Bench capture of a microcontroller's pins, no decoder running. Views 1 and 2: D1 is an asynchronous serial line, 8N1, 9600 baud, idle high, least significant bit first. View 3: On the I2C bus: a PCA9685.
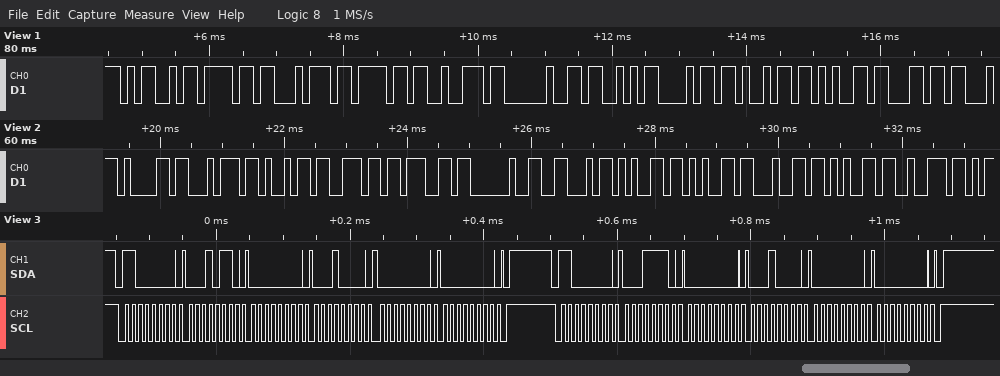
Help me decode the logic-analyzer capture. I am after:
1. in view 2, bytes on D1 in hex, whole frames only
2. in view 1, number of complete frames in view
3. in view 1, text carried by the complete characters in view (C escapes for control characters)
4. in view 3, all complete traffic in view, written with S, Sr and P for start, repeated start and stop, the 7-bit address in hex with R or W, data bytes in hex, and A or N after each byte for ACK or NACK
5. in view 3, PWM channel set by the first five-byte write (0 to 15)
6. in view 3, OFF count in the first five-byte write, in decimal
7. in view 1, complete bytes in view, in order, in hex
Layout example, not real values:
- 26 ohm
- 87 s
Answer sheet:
- 0x61 0x74 0x69 0x6E 0x67 0x20 0x46 0x65 0x65 0x64 0x65 0x72
- 11
- "Motor Shiel"
- S 60W A 16 A 00 A 10 A 00 A 00 A P S 60W A 1E A 00 A 10 A 00 A 00 A P
- 4
- 0
- 0x4D 0x6F 0x74 0x6F 0x72 0x20 0x53 0x68 0x69 0x65 0x6C
